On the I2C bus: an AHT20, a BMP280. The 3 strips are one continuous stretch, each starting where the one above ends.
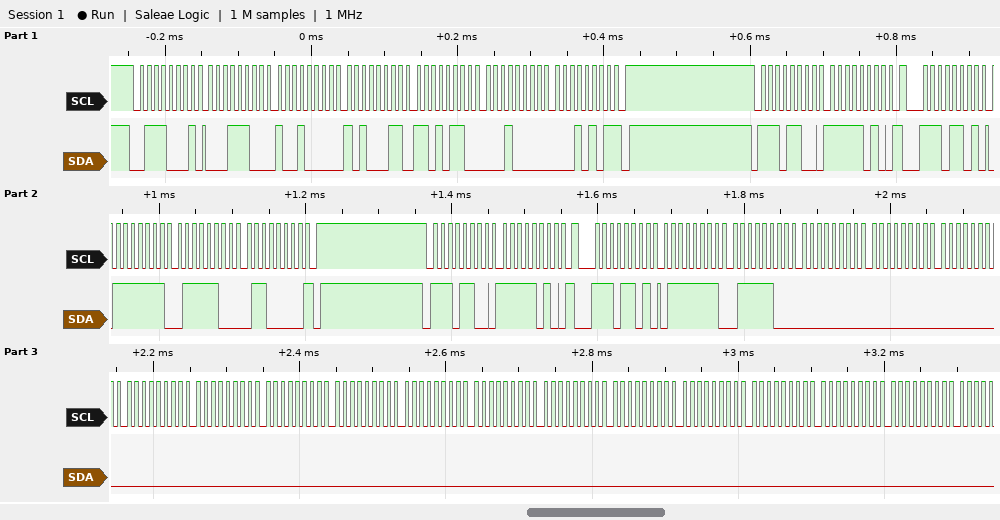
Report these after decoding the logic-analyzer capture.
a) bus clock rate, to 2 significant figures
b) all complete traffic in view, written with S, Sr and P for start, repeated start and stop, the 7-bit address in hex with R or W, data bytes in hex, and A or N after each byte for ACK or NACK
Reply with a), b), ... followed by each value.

a) 100 kHz
b) S 38R A 1C A 90 A A3 A D6 A 10 A 15 N P S 76W A FA A Sr 76R A 7F A 7C A 60 N P S 76W A FA A Sr 76R A 7F A 7C A 00 A 00 A 00 A 00 A 00 A 00 A 00 A 00 A 00 A 00 A 00 A 00 A 00 A 00 A 00 A
